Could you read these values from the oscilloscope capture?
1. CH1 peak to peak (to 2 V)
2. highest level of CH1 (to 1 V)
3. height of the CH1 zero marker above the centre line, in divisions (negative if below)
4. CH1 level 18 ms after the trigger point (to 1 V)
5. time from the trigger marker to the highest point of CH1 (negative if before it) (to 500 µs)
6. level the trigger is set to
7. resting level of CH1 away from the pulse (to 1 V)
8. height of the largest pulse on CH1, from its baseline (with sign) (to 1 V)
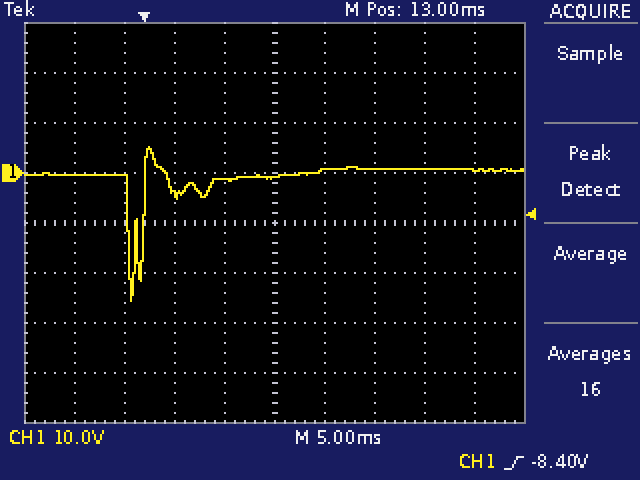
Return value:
30 V
5 V
+1.0 div
1 V
+500 µs
-8.40 V
0 V
-26 V
